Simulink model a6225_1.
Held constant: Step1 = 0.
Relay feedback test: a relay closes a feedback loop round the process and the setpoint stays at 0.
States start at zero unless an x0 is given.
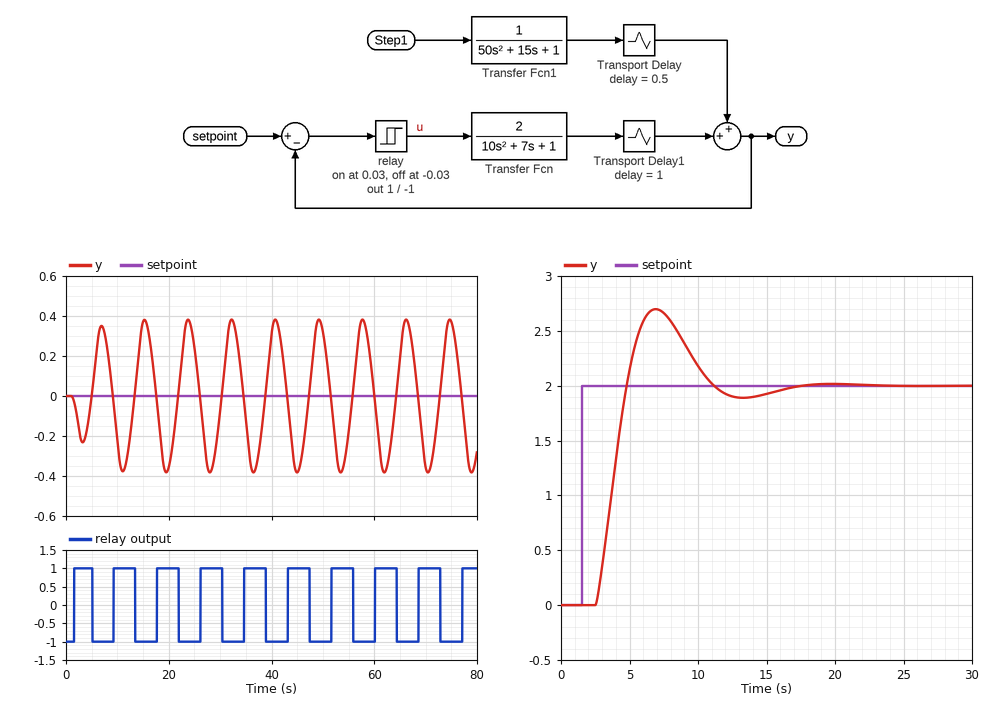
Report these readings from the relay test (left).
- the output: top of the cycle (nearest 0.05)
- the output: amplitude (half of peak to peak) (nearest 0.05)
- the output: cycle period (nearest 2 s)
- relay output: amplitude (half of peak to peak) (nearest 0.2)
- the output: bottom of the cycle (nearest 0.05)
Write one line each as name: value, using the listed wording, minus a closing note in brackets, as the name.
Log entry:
the output: top of the cycle: 0.40
the output: amplitude (half of peak to peak): 0.40
the output: cycle period: 8 s
relay output: amplitude (half of peak to peak): 1.0
the output: bottom of the cycle: -0.40
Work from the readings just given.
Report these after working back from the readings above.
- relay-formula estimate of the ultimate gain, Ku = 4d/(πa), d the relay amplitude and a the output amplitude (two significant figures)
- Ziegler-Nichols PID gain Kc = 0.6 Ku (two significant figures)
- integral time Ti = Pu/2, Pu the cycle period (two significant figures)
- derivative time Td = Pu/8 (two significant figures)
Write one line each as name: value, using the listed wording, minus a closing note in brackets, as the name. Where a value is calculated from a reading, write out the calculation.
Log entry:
relay-formula estimate of the ultimate gain, Ku = 4d/(πa), d the relay amplitude and a the output amplitude: 4 × 1 / (π × 0.4) = 3.2
Ziegler-Nichols PID gain Kc = 0.6 Ku: 0.6 × 3.2 = 1.9
integral time Ti = Pu/2, Pu the cycle period: 8 / 2 = 4.0 s
derivative time Td = Pu/8: 8 / 8 = 1.0 s
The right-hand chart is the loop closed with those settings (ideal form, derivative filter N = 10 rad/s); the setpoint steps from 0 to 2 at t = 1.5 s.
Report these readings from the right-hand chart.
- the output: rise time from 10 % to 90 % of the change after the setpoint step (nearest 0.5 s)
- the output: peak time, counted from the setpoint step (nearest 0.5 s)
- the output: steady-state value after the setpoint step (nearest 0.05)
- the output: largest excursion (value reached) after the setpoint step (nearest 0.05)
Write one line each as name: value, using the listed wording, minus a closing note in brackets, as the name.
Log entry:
the output: rise time from 10 % to 90 % of the change after the setpoint step: 1.5 s
the output: peak time, counted from the setpoint step: 5.5 s
the output: steady-state value after the setpoint step: 2.00
the output: largest excursion (value reached) after the setpoint step: 2.70
